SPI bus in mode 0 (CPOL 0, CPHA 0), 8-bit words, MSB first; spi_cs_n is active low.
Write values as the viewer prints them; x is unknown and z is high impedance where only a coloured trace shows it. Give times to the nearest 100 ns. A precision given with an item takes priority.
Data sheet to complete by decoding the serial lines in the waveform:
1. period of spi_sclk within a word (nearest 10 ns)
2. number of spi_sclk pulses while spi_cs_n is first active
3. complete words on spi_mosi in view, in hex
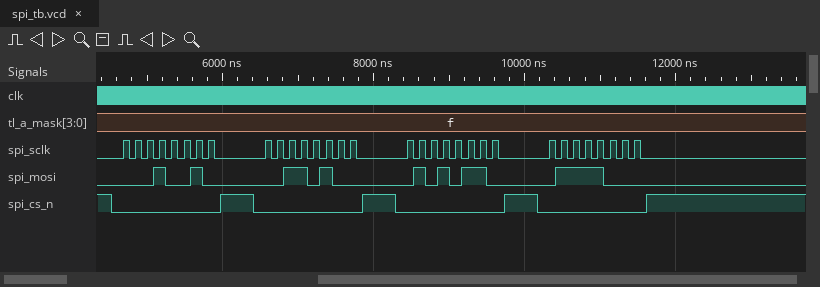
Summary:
160 ns
8
12, 34, 56, 78
